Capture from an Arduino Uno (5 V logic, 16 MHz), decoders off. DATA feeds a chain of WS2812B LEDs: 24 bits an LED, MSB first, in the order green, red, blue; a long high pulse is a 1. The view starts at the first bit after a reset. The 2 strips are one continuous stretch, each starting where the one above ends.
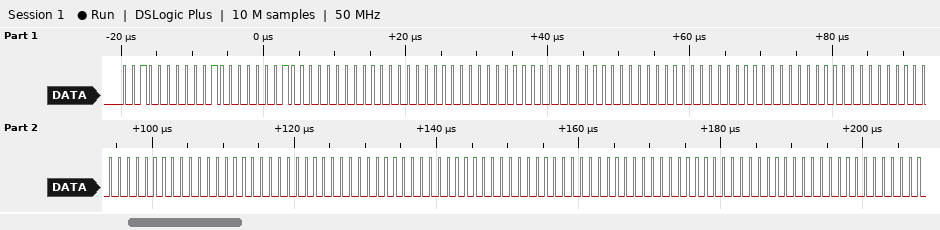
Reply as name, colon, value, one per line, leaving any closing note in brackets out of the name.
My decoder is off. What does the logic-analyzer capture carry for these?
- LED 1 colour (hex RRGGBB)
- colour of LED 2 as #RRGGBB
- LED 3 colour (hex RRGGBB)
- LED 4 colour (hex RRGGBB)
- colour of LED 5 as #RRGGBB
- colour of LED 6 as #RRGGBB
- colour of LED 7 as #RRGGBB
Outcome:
LED 1 colour: #202020
colour of LED 2 as #RRGGBB: #000000
LED 3 colour: #000000
LED 4 colour: #000000
colour of LED 5 as #RRGGBB: #000000
colour of LED 6 as #RRGGBB: #000000
colour of LED 7 as #RRGGBB: #000000
